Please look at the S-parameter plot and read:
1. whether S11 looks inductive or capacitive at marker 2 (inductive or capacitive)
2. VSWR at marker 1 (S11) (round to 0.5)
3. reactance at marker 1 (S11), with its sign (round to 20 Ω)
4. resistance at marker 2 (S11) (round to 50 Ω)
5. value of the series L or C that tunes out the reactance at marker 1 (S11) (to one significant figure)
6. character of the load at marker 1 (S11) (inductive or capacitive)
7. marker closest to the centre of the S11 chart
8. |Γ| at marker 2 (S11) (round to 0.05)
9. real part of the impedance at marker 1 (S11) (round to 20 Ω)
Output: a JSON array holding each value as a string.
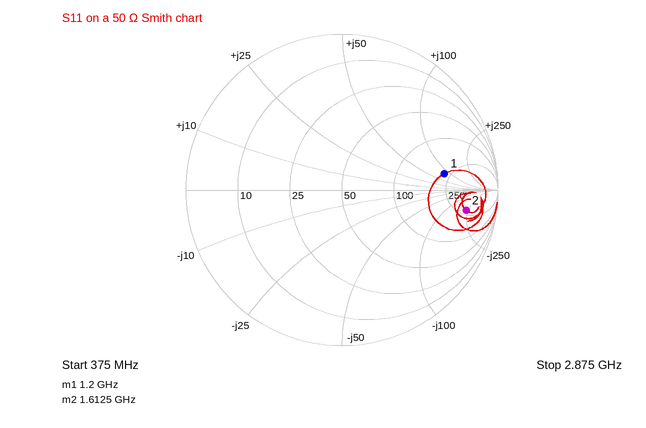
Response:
["capacitive", "5.0", "+80 Ω", "300 Ω", "2 pF", "inductive", "marker 1", "0.80", "220 Ω"]
